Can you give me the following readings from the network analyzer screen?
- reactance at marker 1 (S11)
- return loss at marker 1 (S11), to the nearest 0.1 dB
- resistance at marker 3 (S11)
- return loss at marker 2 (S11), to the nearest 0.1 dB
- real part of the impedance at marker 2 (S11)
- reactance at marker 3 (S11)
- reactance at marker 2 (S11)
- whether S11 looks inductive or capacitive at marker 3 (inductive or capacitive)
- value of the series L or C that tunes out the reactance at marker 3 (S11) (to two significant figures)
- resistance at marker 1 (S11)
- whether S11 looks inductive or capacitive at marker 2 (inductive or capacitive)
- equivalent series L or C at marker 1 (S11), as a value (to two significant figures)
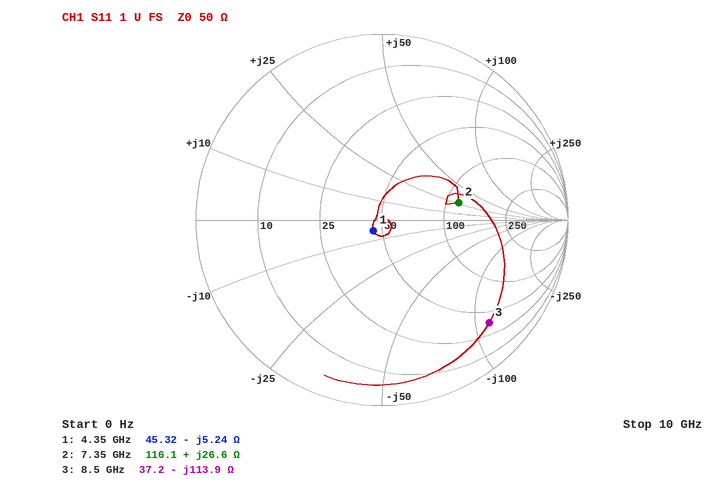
-5.24 Ω
22.7 dB
37.2 Ω
7.5 dB
116.1 Ω
-113.9 Ω
+26.6 Ω
capacitive
2.1 nH
45.32 Ω
inductive
7.0 pF
